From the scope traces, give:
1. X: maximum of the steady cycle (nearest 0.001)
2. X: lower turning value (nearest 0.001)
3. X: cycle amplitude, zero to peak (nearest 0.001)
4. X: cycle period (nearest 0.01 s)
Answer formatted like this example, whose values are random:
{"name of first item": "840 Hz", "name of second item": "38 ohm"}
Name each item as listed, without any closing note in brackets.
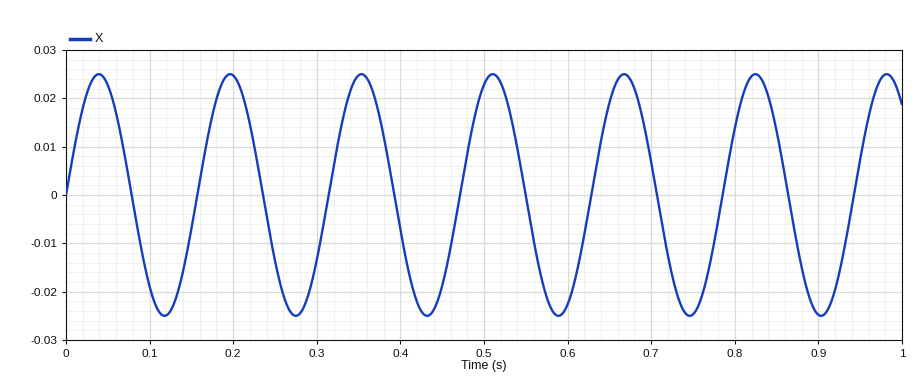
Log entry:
{"X: maximum of the steady cycle": "0.025", "X: lower turning value": "-0.025", "X: cycle amplitude, zero to peak": "0.025", "X: cycle period": "0.16 s"}
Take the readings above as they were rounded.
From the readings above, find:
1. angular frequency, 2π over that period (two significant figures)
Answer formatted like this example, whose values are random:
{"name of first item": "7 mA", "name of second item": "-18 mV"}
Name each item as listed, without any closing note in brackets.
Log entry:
{"angular frequency, 2π over that period": "39 rad/s"}
